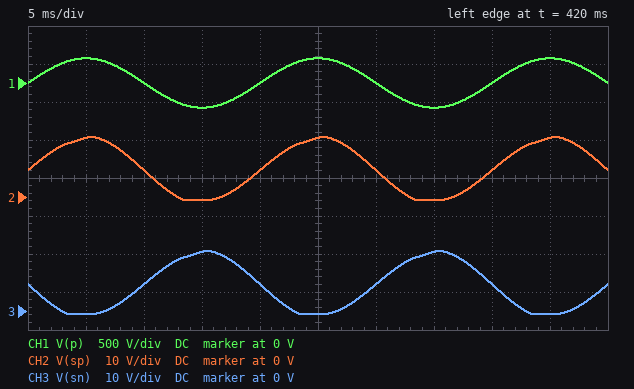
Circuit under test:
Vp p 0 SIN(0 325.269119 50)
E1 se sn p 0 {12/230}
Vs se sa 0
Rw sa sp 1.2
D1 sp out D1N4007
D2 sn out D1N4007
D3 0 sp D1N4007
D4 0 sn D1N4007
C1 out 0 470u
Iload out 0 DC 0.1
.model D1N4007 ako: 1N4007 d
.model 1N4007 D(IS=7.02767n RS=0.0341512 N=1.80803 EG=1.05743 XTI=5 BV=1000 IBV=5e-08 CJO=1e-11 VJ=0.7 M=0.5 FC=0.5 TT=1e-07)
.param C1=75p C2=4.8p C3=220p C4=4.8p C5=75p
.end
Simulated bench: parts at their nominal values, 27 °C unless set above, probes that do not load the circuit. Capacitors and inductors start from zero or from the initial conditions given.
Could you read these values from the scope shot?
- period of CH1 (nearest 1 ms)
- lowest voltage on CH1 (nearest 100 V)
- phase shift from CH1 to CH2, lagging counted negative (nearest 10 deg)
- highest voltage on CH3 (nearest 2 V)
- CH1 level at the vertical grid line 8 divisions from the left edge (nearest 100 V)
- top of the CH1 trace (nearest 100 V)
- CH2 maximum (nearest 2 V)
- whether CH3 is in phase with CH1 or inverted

20 ms
-300 V
0 deg
16 V
0 V
300 V
16 V
inverted
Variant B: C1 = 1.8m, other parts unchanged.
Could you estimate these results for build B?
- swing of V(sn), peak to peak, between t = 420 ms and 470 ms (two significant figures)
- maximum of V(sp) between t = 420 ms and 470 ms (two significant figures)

16 V
15 V
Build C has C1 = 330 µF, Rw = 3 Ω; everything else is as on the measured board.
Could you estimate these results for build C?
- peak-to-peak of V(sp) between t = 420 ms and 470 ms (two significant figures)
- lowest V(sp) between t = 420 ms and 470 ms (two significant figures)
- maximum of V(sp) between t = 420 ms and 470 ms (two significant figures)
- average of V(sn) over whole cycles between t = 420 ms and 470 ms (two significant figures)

16 V
-860 mV
15 V
6.7 V
